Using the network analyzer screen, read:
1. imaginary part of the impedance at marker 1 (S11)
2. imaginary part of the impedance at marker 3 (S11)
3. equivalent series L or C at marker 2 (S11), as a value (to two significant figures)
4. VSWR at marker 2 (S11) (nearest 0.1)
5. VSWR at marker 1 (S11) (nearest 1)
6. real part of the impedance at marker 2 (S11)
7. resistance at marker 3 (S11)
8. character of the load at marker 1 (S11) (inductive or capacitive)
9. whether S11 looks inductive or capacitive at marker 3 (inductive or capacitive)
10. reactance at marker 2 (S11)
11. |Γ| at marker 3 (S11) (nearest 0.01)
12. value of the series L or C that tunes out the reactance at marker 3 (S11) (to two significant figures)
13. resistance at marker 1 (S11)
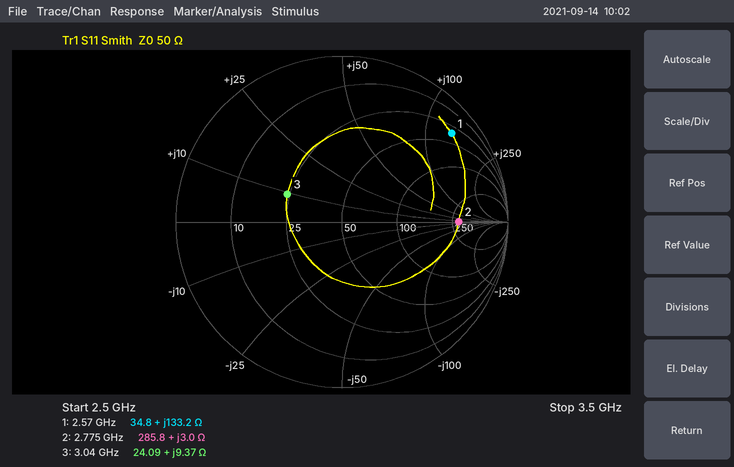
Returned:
+133.2 Ω
+9.37 Ω
170 pH
5.7
12
285.8 Ω
24.09 Ω
inductive
inductive
+3.0 Ω
0.37
5.6 pF
34.8 Ω
